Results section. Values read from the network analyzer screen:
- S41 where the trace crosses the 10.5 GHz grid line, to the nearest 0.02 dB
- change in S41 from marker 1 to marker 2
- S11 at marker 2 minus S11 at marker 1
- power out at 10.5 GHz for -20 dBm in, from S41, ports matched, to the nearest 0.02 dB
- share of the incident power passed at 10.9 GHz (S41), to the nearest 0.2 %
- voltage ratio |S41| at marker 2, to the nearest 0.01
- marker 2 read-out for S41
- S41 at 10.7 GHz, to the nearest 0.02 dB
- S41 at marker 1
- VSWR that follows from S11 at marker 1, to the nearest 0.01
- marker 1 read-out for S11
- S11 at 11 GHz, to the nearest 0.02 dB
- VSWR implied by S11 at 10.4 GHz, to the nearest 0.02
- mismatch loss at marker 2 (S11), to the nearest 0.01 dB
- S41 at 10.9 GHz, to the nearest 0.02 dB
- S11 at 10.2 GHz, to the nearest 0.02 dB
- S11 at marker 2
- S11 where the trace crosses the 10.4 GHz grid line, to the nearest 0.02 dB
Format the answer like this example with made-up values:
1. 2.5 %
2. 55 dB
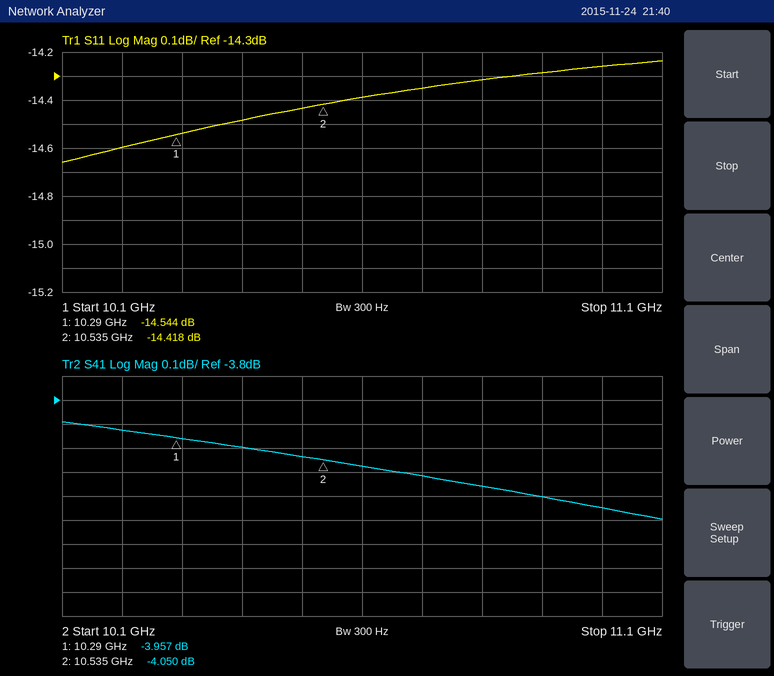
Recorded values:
1. -4.04 dB
2. -0.093 dB
3. 0.126 dB
4. -24.04 dBm
5. 38.0 %
6. 0.63
7. -4.050 dB
8. -4.12 dB
9. -3.957 dB
10. 1.46
11. -14.544 dB
12. -14.26 dB
13. 1.46
14. 0.16 dB
15. -4.20 dB
16. -14.60 dB
17. -14.418 dB
18. -14.48 dB
